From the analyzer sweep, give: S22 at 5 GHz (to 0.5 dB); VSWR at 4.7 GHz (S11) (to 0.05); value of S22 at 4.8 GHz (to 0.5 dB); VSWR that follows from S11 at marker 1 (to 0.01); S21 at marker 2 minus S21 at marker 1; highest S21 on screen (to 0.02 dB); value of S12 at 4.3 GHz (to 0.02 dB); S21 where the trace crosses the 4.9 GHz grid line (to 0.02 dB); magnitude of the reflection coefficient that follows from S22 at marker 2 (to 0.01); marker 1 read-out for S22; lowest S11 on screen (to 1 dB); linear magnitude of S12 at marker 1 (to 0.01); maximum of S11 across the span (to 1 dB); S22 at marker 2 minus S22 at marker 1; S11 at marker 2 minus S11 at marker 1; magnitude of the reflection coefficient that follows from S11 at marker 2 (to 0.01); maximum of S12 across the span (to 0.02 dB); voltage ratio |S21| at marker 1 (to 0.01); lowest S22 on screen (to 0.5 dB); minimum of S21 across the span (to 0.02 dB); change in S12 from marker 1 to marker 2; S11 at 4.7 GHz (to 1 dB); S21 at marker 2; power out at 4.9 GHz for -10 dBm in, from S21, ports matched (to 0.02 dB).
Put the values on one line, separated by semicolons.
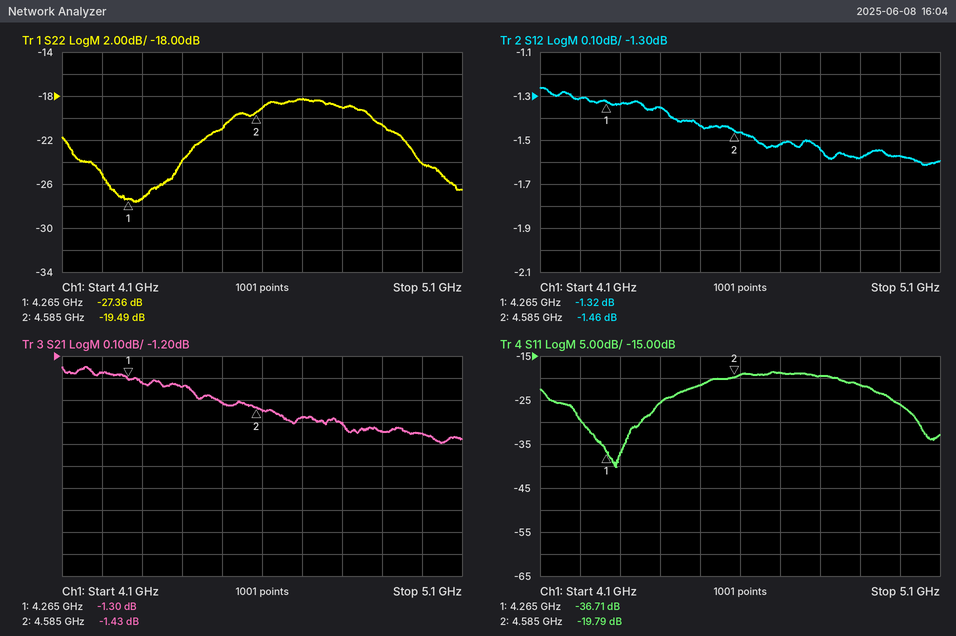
-24.0 dB; 1.25; -19.0 dB; 1.03; -0.13 dB; -1.24 dB; -1.34 dB; -1.54 dB; 0.11; -27.36 dB; -40 dB; 0.86; -19 dB; 7.87 dB; 16.92 dB; 0.10; -1.26 dB; 0.86; -27.5 dB; -1.60 dB; -0.14 dB; -19 dB; -1.43 dB; -11.54 dBm
